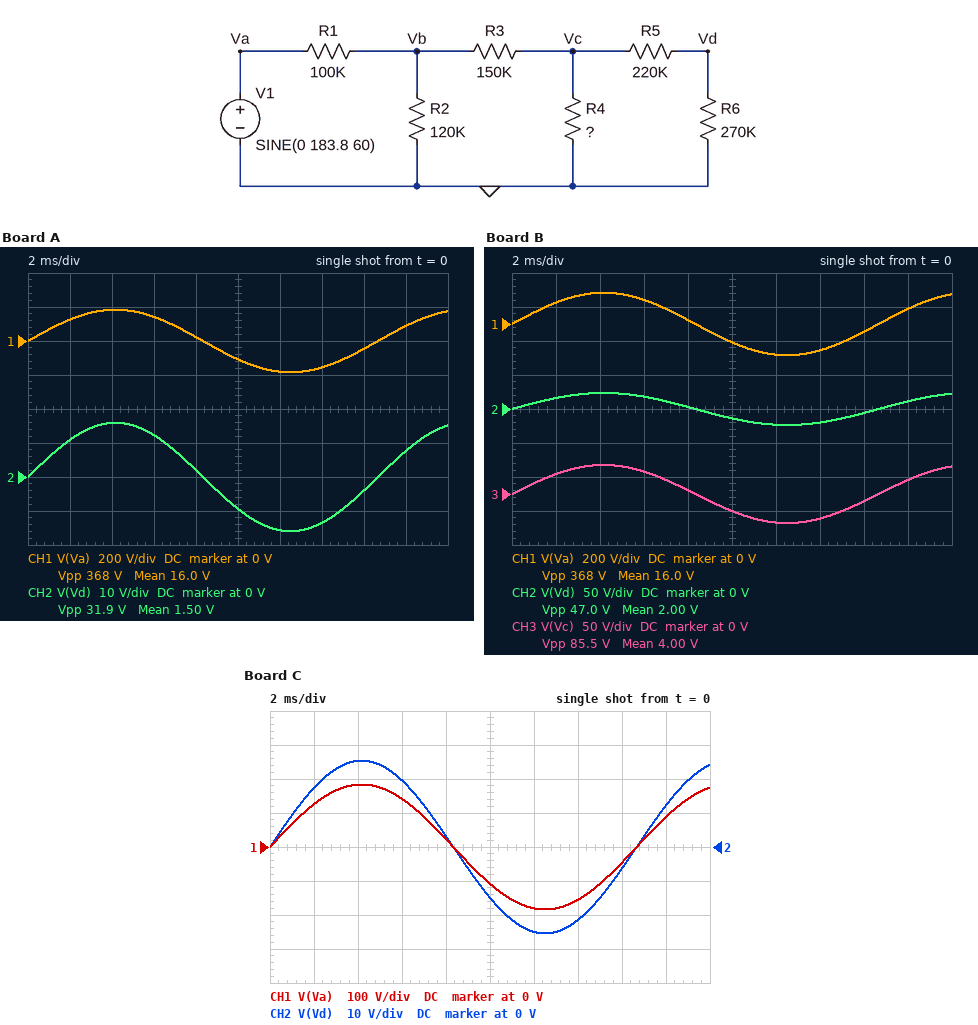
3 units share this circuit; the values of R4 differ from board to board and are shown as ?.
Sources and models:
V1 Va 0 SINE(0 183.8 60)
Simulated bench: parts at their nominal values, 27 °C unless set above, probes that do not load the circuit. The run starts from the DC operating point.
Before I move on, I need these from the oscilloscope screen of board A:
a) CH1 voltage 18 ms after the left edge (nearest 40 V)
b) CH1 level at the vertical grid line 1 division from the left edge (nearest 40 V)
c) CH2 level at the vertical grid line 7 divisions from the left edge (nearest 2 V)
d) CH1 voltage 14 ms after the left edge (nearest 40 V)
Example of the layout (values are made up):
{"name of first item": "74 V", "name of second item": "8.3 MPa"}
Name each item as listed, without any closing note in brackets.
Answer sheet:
{"CH1 voltage 18 ms after the left edge": "80 V", "CH1 level at the vertical grid line 1 division from the left edge": "120 V", "CH2 level at the vertical grid line 7 divisions from the left edge": "-14 V", "CH1 voltage 14 ms after the left edge": "-160 V"}
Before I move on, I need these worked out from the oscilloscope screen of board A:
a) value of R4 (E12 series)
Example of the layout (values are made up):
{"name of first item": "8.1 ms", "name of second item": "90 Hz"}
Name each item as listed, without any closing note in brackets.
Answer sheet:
{"value of R4": "100 kΩ"}
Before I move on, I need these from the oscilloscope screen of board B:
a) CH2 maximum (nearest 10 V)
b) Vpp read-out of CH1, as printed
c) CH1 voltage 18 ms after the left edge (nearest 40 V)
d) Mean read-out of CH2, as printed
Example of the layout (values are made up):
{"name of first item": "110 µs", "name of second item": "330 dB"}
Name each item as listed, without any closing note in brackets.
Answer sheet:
{"CH2 maximum": "20 V", "Vpp read-out of CH1, as printed": "368 V", "CH1 voltage 18 ms after the left edge": "80 V", "Mean read-out of CH2, as printed": "2.00 V"}
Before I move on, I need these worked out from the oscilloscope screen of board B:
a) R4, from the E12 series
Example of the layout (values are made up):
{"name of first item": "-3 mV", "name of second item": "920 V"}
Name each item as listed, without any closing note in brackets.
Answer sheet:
{"R4, from the E12 series": "220 kΩ"}
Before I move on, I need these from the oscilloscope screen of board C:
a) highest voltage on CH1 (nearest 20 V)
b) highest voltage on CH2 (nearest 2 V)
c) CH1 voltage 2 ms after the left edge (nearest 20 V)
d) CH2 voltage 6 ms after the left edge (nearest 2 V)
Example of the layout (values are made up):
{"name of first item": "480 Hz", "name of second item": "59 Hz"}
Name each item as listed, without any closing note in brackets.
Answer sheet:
{"highest voltage on CH1": "180 V", "highest voltage on CH2": "26 V", "CH1 voltage 2 ms after the left edge": "120 V", "CH2 voltage 6 ms after the left edge": "20 V"}
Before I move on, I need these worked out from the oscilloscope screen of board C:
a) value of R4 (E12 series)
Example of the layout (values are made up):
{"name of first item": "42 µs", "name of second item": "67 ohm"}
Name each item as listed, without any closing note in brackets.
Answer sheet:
{"value of R4": "270 kΩ"}
